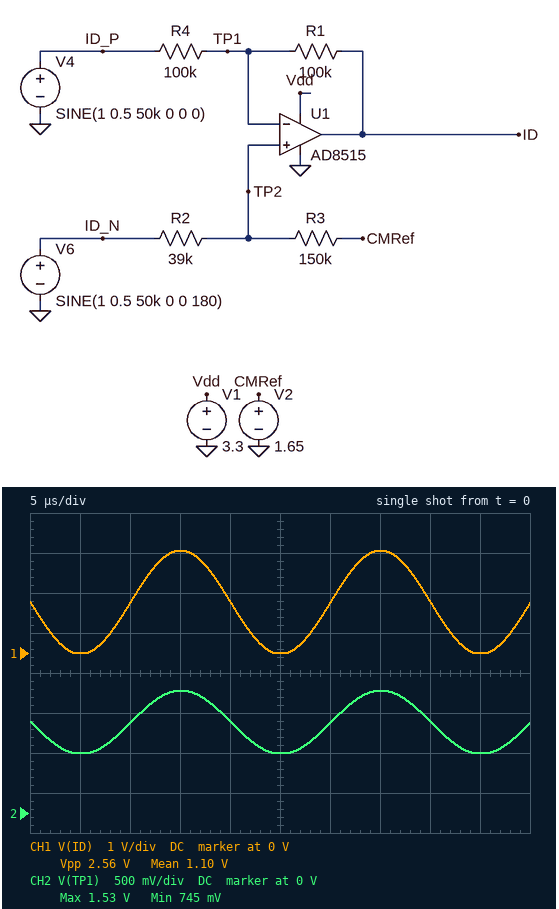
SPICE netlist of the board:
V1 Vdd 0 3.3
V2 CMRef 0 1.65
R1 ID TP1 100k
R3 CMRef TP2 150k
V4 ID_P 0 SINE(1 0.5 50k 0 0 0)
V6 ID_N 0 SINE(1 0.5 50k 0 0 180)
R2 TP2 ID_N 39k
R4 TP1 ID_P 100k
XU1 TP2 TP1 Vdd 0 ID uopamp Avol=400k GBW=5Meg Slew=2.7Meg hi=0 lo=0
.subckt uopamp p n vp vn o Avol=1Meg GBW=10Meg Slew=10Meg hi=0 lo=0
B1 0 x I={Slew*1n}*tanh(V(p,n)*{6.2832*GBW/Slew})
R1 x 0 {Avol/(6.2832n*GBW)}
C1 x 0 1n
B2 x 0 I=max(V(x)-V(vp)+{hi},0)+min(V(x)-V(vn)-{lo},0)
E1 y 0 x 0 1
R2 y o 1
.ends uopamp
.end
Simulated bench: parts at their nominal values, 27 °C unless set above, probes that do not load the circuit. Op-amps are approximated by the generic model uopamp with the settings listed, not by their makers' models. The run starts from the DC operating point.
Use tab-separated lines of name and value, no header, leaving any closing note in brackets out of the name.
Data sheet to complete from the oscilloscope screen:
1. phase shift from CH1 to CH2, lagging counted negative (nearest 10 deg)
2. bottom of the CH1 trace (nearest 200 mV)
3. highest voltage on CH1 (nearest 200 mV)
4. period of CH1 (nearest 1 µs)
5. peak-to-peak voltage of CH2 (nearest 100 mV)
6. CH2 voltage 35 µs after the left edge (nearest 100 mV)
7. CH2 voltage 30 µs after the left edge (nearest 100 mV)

phase shift from CH1 to CH2, lagging counted negative	0 deg
bottom of the CH1 trace	0 V
highest voltage on CH1	2.6 V
period of CH1	20 µs
peak-to-peak voltage of CH2	800 mV
CH2 voltage 35 µs after the left edge	1.5 V
CH2 voltage 30 µs after the left edge	1.1 V
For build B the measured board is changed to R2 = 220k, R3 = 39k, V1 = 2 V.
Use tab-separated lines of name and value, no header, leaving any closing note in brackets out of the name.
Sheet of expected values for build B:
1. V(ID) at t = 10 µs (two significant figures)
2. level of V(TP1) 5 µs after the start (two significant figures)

V(ID) at t = 10 µs	2.0 V
level of V(TP1) 5 µs after the start	1.5 V
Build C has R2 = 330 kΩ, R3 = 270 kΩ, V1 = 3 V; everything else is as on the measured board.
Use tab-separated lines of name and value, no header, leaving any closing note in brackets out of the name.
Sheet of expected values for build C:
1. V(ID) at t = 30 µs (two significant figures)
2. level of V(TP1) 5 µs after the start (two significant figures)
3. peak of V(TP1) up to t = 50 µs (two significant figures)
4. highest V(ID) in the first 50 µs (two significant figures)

V(ID) at t = 30 µs	1.7 V
level of V(TP1) 5 µs after the start	1.1 V
peak of V(TP1) up to t = 50 µs	1.6 V
highest V(ID) in the first 50 µs	2.7 V
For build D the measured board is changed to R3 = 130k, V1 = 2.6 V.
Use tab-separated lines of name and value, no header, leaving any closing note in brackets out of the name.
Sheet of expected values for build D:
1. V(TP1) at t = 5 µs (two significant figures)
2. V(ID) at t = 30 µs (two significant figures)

V(TP1) at t = 5 µs	770 mV
V(ID) at t = 30 µs	1.3 V
